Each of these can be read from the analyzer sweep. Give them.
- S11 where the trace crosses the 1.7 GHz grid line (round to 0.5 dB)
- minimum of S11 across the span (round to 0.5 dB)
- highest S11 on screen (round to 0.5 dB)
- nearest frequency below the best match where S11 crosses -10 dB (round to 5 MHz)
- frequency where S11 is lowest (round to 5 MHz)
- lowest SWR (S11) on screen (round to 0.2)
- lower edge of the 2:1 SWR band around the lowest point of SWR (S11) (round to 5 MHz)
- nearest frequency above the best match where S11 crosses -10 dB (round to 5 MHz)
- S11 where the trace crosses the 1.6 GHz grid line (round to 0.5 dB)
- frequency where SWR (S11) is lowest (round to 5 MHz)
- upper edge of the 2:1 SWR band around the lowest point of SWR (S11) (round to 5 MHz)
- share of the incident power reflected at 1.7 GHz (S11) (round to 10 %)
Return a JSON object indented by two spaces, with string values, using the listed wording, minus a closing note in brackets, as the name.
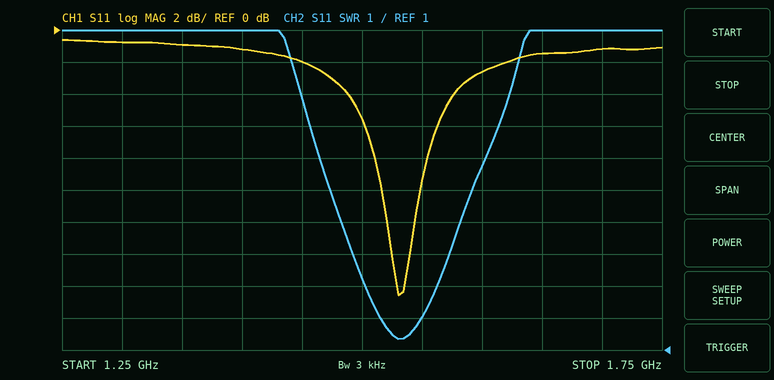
{
  "S11 where the trace crosses the 1.7 GHz grid line": "-1.0 dB",
  "minimum of S11 across the span": "-16.5 dB",
  "highest S11 on screen": "-0.5 dB",
  "nearest frequency below the best match where S11 crosses -10 dB": "1.515 GHz",
  "frequency where S11 is lowest": "1.530 GHz",
  "lowest SWR (S11) on screen": "1.4",
  "lower edge of the 2:1 SWR band around the lowest point of SWR (S11)": "1.515 GHz",
  "nearest frequency above the best match where S11 crosses -10 dB": "1.550 GHz",
  "S11 where the trace crosses the 1.6 GHz grid line": "-2.5 dB",
  "frequency where SWR (S11) is lowest": "1.530 GHz",
  "upper edge of the 2:1 SWR band around the lowest point of SWR (S11)": "1.550 GHz",
  "share of the incident power reflected at 1.7 GHz (S11)": "80 %"
}
